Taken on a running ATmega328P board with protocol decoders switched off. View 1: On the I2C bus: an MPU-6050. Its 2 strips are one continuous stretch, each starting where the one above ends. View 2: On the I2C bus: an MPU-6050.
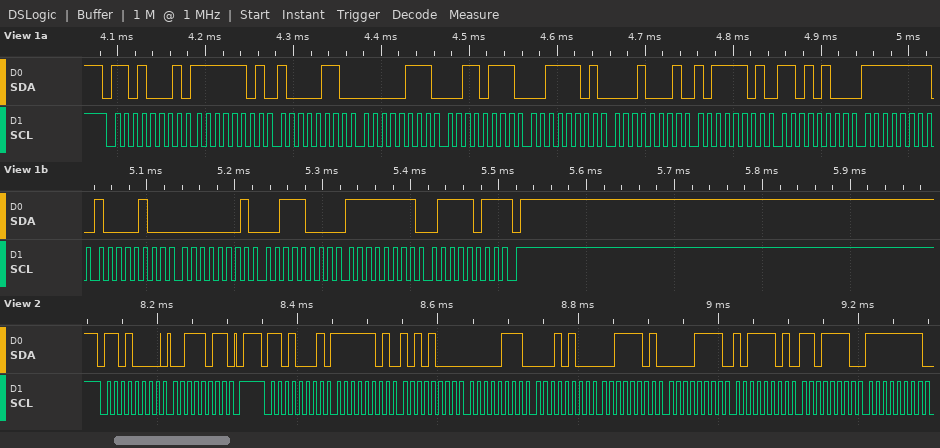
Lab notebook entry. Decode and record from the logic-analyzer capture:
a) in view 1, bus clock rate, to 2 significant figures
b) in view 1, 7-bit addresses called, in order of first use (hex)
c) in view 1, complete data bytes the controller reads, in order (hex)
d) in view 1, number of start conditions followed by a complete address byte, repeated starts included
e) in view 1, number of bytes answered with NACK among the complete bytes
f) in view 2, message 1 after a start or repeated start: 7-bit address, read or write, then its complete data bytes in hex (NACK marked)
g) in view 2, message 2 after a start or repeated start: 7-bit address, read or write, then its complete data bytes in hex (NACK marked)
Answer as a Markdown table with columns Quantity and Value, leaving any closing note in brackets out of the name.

| Quantity | Value |
|---|---|
| in view 1, bus clock rate, to 2 significant figures | 100 kHz |
| in view 1, 7-bit addresses called, in order of first use | 0x68 |
| in view 1, complete data bytes the controller reads, in order | FD 86 07 37 3D 11 BD D4 FF 84 01 38 FF 7B |
| in view 1, number of start conditions followed by a complete address byte, repeated starts included | 1 |
| in view 1, number of bytes answered with NACK among the complete bytes | 1 |
| in view 2, message 1 after a start or repeated start: 7-bit address, read or write, then its complete data bytes in hex | 0x68 write: 3B |
| in view 2, message 2 after a start or repeated start: 7-bit address, read or write, then its complete data bytes in hex | 0x68 read: FD A8 07 14 3D 0F BD DE FF |
